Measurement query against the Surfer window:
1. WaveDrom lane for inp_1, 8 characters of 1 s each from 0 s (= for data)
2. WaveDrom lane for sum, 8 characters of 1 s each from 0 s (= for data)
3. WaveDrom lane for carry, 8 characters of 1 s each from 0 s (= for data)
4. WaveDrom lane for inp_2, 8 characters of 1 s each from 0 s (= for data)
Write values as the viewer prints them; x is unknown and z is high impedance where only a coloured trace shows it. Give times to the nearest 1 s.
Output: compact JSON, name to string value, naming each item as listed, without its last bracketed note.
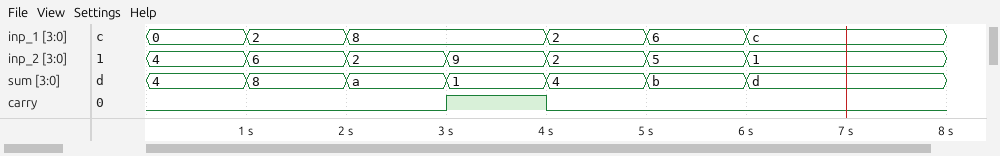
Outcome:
{"WaveDrom lane for inp_1, 8 characters of 1 s each from 0 s": "{name: 'inp_1', wave: '===.===.', data: '0 2 8 2 6 c'}", "WaveDrom lane for sum, 8 characters of 1 s each from 0 s": "{name: 'sum', wave: '=======.', data: '4 8 a 1 4 b d'}", "WaveDrom lane for carry, 8 characters of 1 s each from 0 s": "{name: 'carry', wave: '0..10...'}", "WaveDrom lane for inp_2, 8 characters of 1 s each from 0 s": "{name: 'inp_2', wave: '=======.', data: '4 6 2 9 2 5 1'}"}
